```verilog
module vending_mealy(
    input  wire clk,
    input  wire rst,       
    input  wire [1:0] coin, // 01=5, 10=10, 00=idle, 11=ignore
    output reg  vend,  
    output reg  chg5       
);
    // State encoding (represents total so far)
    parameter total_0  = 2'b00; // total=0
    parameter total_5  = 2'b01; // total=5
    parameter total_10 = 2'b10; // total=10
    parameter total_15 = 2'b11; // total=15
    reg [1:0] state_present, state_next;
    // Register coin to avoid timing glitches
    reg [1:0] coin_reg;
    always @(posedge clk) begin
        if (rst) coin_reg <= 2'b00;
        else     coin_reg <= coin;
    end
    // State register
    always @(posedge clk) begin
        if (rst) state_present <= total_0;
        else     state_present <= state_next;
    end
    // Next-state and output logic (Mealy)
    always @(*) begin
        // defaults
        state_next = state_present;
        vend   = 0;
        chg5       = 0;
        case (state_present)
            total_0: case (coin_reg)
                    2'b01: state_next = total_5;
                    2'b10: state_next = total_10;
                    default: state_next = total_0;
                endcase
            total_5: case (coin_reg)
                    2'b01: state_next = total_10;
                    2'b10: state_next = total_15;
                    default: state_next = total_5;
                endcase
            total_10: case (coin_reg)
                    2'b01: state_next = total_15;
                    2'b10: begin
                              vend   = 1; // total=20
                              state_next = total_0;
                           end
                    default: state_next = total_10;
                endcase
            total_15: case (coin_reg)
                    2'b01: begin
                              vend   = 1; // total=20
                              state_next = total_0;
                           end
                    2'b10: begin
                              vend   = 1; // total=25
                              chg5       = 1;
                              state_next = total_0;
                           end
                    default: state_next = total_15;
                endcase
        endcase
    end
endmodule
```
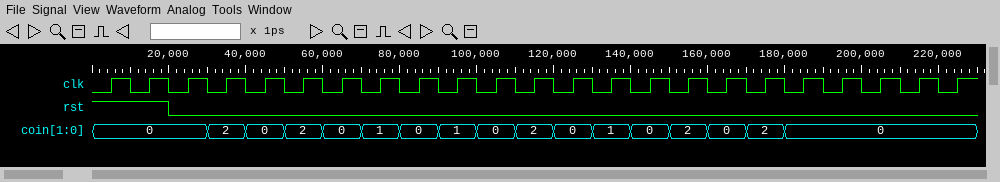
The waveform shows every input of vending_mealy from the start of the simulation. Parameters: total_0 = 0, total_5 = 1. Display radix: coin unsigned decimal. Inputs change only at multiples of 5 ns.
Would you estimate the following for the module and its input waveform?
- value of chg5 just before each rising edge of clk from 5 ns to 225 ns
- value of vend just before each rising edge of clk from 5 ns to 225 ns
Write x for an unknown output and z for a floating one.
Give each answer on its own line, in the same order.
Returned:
x 0 0 0 0 0 0 0 0 0 0 0 0 0 0 0 0 0 1 0 0 0 0
x 0 0 0 0 0 1 0 0 0 0 0 1 0 0 0 0 0 1 0 0 0 0
